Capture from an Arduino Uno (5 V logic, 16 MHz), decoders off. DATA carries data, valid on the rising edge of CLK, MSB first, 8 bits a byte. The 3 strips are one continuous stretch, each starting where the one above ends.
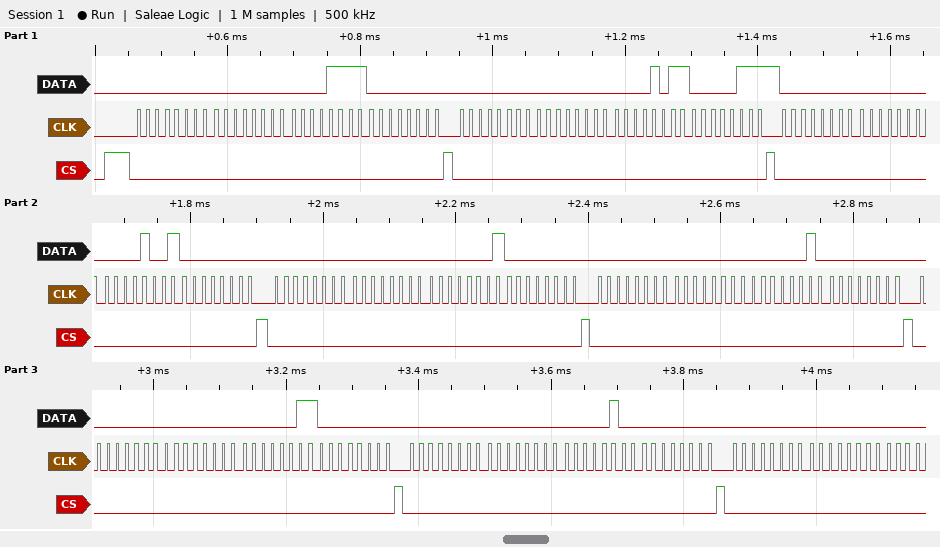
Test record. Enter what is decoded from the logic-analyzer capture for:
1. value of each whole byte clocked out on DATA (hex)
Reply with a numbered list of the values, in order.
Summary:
1. 00 00 0F 00 00 00 0B 07 00 00 09 00 00 00 01 00 00 00 02 00 00 00 03 00 00 00 04 00 00 00
